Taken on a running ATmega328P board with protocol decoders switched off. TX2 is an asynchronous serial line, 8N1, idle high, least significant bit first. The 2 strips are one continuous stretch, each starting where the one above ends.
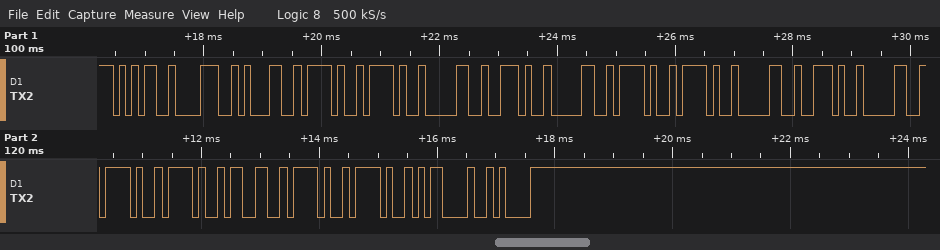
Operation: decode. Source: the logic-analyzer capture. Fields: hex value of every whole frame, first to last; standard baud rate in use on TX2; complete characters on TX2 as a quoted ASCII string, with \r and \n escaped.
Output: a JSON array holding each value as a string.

["35 38 31 2F 2F 30 2E 30 2F 2F 30 2E 30 2F 2F 33 2F 2F 0D 0A", "9600 baud", "\"581//0.0//0.0//3//\\r\\n\""]
